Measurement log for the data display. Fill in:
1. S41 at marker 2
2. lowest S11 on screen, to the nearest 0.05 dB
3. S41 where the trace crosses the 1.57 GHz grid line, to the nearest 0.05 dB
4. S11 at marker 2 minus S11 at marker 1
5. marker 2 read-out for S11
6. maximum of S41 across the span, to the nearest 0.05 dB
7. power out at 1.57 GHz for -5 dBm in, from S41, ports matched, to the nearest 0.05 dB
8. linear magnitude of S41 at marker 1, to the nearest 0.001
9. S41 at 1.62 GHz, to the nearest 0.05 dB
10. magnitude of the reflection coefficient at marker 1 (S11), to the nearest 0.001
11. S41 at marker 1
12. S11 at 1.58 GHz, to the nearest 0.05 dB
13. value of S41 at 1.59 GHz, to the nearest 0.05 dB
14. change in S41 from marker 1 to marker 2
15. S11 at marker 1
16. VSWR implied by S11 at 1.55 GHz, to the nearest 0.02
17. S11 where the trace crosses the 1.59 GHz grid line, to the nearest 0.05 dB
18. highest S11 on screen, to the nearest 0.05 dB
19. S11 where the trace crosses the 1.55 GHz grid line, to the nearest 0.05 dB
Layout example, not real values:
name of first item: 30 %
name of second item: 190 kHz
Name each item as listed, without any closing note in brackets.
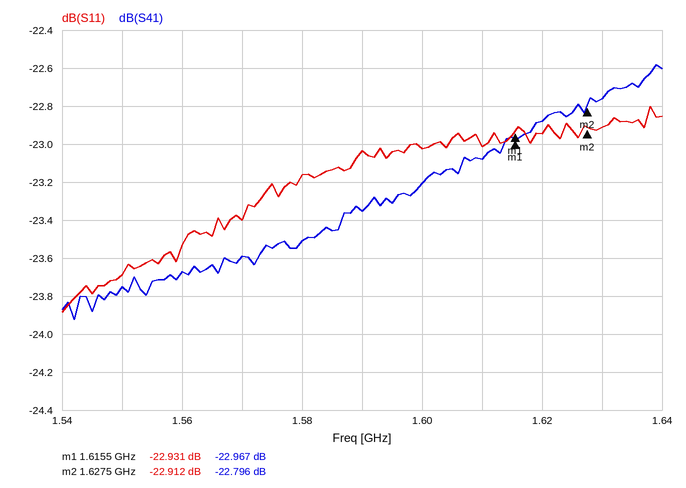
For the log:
S41 at marker 2: -22.796 dB
lowest S11 on screen, to the nearest 0.05 dB: -23.90 dB
S41 where the trace crosses the 1.57 GHz grid line, to the nearest 0.05 dB: -23.60 dB
S11 at marker 2 minus S11 at marker 1: 0.019 dB
marker 2 read-out for S11: -22.912 dB
maximum of S41 across the span, to the nearest 0.05 dB: -22.60 dB
power out at 1.57 GHz for -5 dBm in, from S41, ports matched, to the nearest 0.05 dB: -28.60 dBm
linear magnitude of S41 at marker 1, to the nearest 0.001: 0.071
S41 at 1.62 GHz, to the nearest 0.05 dB: -22.90 dB
magnitude of the reflection coefficient at marker 1 (S11), to the nearest 0.001: 0.071
S41 at marker 1: -22.967 dB
S11 at 1.58 GHz, to the nearest 0.05 dB: -23.15 dB
value of S41 at 1.59 GHz, to the nearest 0.05 dB: -23.35 dB
change in S41 from marker 1 to marker 2: 0.171 dB
S11 at marker 1: -22.931 dB
VSWR implied by S11 at 1.55 GHz, to the nearest 0.02: 1.14
S11 where the trace crosses the 1.59 GHz grid line, to the nearest 0.05 dB: -23.05 dB
highest S11 on screen, to the nearest 0.05 dB: -22.80 dB
S11 where the trace crosses the 1.55 GHz grid line, to the nearest 0.05 dB: -23.70 dB
